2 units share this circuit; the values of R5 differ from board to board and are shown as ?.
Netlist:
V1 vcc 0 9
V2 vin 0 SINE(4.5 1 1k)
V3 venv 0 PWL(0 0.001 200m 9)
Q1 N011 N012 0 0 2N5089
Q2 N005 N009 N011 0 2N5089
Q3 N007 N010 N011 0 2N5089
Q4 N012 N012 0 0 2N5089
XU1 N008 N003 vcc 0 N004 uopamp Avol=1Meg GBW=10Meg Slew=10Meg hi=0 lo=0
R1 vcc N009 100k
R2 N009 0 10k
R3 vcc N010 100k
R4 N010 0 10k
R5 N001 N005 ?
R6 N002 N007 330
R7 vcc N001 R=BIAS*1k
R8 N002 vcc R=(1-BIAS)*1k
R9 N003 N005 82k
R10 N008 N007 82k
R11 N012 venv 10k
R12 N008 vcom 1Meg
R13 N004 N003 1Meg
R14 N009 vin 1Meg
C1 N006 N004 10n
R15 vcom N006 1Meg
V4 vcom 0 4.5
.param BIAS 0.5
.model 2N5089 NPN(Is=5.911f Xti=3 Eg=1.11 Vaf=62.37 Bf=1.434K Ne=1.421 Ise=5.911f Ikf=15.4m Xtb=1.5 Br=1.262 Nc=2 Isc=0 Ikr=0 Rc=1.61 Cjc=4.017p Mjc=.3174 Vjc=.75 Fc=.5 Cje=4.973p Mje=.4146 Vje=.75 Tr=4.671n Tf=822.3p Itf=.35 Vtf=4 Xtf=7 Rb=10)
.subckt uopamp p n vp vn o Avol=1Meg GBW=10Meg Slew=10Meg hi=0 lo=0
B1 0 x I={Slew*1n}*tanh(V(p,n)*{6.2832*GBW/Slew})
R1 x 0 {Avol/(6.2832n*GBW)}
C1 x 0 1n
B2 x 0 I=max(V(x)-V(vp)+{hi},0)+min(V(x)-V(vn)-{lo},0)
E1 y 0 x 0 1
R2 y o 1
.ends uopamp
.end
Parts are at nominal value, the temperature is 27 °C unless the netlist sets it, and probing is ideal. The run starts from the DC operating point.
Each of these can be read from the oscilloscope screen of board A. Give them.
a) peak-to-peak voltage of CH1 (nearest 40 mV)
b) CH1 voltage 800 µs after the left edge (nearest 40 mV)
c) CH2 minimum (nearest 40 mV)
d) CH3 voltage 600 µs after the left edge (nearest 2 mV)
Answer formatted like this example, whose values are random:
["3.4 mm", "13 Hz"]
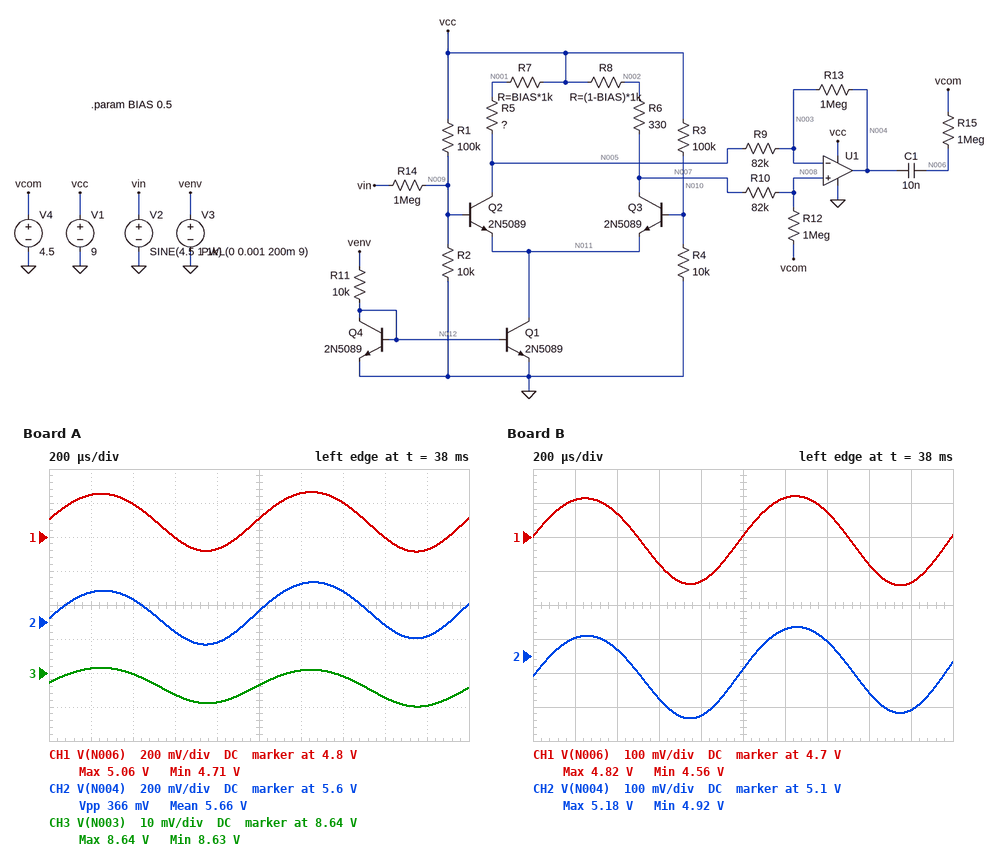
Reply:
["360 mV", "4.72 V", "5.48 V", "8.634 V"]
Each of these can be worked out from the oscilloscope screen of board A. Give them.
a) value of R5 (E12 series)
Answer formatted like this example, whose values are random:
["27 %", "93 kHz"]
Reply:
["820 Ω"]
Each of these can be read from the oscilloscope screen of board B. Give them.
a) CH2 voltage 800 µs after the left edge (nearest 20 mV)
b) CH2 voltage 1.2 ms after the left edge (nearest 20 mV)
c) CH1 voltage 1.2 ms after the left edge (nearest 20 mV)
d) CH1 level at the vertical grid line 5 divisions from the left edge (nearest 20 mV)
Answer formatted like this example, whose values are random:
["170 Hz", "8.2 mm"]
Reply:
["4.92 V", "5.18 V", "4.82 V", "4.70 V"]
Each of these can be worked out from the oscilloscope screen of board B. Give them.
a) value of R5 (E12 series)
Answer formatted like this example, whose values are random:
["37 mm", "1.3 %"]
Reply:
["270 Ω"]
